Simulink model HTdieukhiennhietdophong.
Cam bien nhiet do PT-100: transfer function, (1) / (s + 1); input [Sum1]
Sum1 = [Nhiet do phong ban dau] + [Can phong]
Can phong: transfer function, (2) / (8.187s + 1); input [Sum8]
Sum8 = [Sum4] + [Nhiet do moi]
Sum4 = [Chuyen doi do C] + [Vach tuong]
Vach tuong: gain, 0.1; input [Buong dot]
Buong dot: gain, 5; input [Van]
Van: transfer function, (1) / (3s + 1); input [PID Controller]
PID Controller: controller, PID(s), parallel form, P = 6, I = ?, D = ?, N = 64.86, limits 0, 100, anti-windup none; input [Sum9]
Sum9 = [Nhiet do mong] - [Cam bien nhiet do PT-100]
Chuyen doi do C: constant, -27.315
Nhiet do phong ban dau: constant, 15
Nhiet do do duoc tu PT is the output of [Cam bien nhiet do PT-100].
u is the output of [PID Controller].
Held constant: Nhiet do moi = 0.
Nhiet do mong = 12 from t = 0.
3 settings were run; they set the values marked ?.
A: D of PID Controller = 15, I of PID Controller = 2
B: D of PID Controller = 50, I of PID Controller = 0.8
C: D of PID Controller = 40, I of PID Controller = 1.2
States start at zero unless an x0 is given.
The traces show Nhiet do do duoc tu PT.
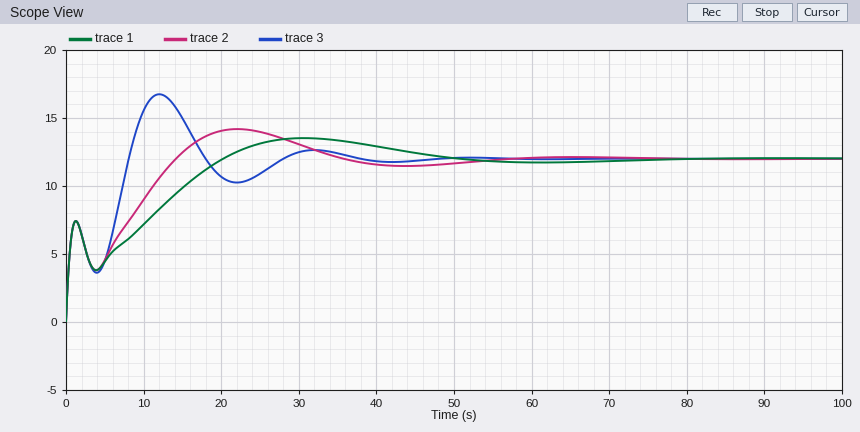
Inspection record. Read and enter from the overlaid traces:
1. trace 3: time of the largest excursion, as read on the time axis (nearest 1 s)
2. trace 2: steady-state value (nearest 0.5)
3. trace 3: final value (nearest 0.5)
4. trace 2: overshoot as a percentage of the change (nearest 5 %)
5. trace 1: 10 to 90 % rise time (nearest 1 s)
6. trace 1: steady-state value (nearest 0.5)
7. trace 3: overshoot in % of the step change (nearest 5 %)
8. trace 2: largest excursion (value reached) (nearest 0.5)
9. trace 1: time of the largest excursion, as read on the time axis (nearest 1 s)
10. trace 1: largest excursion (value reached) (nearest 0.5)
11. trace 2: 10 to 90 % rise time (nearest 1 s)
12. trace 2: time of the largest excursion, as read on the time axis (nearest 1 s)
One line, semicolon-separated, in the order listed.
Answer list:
12 s; 12.0; 12.0; 20 %; 17 s; 12.0; 40 %; 14.0; 31 s; 13.5; 12 s; 22 s
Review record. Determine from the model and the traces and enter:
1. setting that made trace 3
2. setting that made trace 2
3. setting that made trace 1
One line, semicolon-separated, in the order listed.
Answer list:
A; C; B
